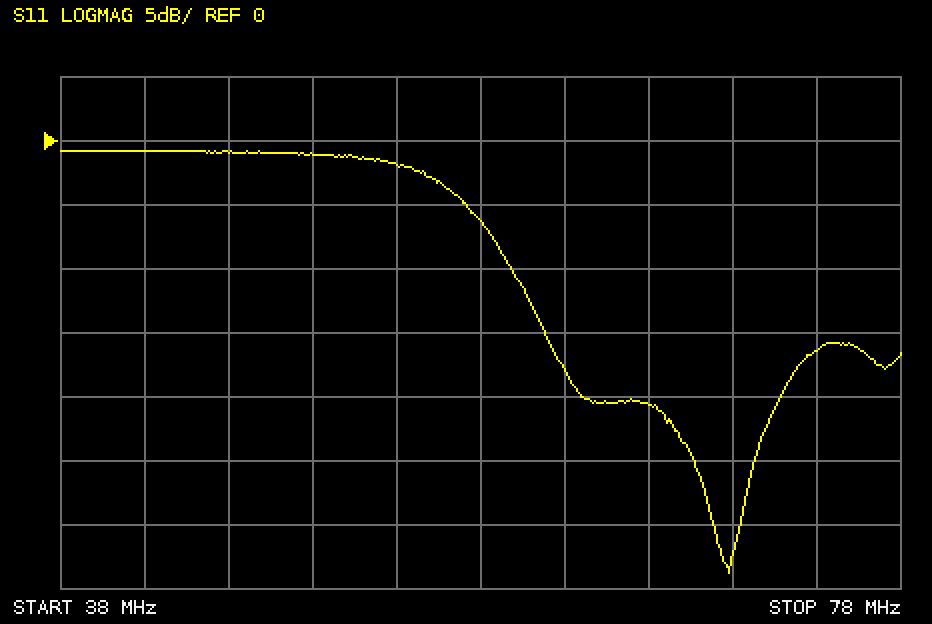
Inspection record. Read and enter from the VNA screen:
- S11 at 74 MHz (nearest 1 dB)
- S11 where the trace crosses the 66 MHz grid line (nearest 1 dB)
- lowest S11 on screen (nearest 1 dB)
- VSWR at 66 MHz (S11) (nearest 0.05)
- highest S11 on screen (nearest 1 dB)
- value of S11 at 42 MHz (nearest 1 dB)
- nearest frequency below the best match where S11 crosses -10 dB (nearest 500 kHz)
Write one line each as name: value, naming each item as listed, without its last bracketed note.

S11 at 74 MHz: -16 dB
S11 where the trace crosses the 66 MHz grid line: -21 dB
lowest S11 on screen: -34 dB
VSWR at 66 MHz (S11): 1.20
highest S11 on screen: -1 dB
value of S11 at 42 MHz: -1 dB
nearest frequency below the best match where S11 crosses -10 dB: 59.5 MHz
